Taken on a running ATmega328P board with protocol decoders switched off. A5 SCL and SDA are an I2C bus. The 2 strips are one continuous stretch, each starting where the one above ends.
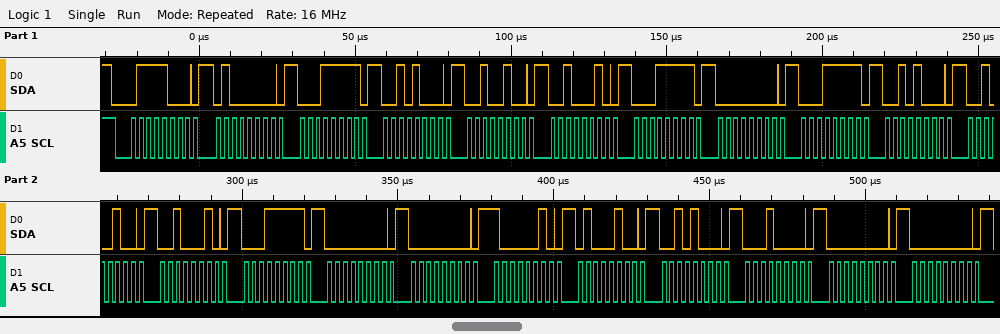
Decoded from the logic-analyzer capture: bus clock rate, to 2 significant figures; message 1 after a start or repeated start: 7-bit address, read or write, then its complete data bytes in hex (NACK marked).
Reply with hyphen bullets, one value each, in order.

- 400 kHz
- 0x3C write: 40 1F 28 24 22 1F 00 1F 28 24 22 1F 00 00 82 44 28 10 00 00
